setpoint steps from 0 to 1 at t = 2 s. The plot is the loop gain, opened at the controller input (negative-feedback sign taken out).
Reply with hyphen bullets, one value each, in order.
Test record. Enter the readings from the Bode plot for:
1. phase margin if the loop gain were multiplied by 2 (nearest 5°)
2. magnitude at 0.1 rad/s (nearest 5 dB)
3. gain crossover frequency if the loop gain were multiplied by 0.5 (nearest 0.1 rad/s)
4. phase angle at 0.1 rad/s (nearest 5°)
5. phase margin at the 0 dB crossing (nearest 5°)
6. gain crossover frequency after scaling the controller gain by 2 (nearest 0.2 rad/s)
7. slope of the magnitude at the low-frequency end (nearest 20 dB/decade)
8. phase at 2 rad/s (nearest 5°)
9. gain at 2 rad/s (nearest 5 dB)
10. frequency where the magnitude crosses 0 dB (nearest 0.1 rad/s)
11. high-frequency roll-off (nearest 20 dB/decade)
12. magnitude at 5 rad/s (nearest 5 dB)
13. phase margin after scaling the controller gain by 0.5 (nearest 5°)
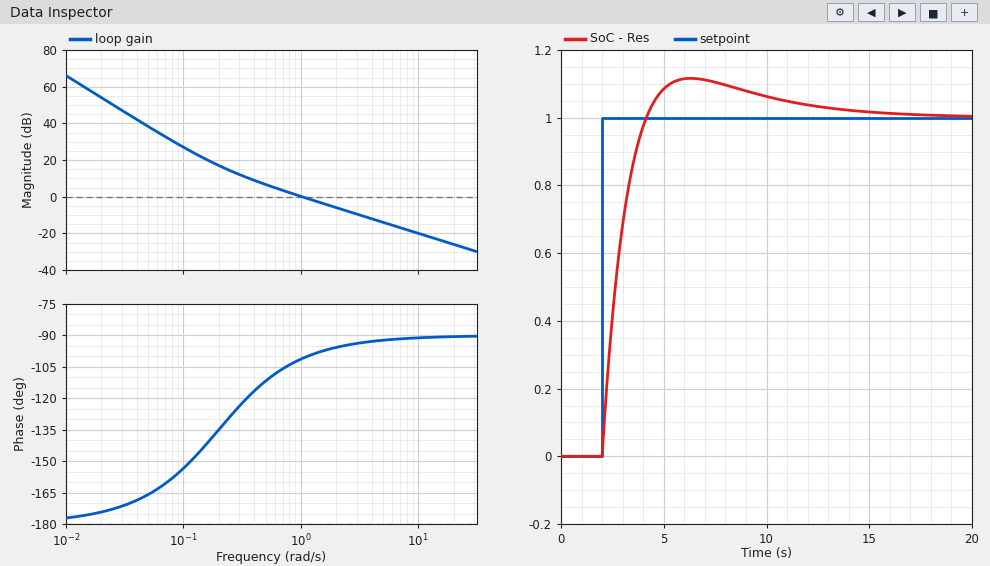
- 85°
- 25 dB
- 0.5 rad/s
- -155°
- 80°
- 2.0 rad/s
- -40 dB/decade
- -95°
- -5 dB
- 1.0 rad/s
- -20 dB/decade
- -15 dB
- 70°
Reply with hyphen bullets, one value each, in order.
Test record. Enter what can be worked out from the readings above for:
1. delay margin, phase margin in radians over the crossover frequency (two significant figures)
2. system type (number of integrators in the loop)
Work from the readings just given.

- 1.4 s
- 2
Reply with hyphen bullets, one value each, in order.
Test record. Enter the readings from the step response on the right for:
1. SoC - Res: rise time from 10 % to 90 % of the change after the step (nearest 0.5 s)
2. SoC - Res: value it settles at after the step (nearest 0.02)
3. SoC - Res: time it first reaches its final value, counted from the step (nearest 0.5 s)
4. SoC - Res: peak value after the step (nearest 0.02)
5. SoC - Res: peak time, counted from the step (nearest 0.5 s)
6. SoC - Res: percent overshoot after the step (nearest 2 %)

- 1.5 s
- 1.00
- 2.0 s
- 1.12
- 4.5 s
- 12 %
